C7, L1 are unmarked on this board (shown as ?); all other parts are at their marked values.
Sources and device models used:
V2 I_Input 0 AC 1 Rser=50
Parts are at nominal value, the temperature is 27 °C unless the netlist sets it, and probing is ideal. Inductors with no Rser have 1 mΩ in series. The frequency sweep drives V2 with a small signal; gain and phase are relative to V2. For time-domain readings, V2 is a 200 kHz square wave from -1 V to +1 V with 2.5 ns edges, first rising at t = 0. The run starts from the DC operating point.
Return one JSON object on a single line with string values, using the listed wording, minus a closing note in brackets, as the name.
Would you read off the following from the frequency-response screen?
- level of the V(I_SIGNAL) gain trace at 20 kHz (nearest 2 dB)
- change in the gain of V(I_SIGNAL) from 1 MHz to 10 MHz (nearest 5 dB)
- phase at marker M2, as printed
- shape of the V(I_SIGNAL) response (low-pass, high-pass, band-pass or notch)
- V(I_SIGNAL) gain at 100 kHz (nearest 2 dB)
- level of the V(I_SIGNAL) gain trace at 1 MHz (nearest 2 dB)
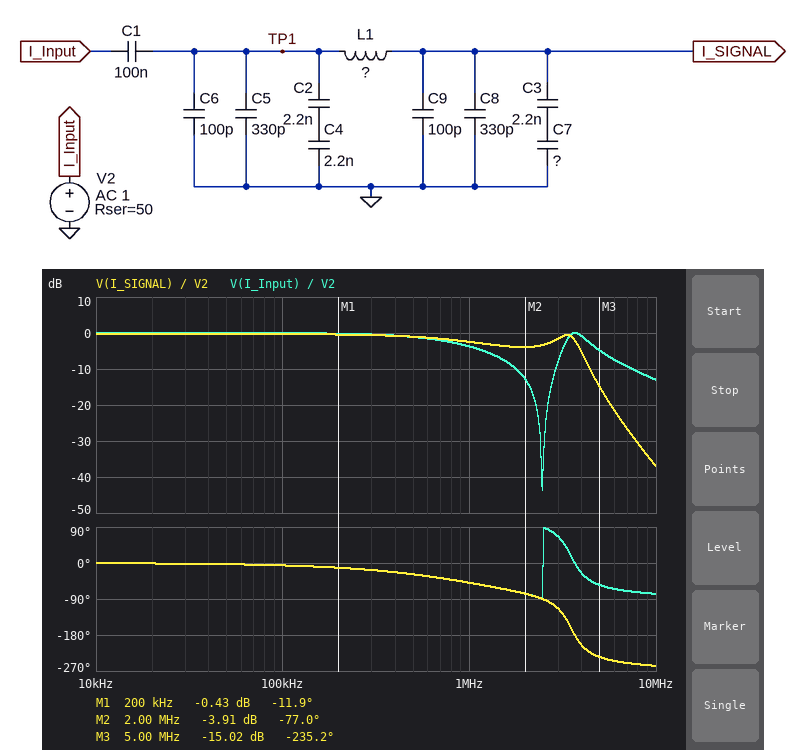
{"level of the V(I_SIGNAL) gain trace at 20 kHz": "0 dB", "change in the gain of V(I_SIGNAL) from 1 MHz to 10 MHz": "-35 dB", "phase at marker M2, as printed": "-77.0 deg", "shape of the V(I_SIGNAL) response": "low-pass", "V(I_SIGNAL) gain at 100 kHz": "0 dB", "level of the V(I_SIGNAL) gain trace at 1 MHz": "-2 dB"}
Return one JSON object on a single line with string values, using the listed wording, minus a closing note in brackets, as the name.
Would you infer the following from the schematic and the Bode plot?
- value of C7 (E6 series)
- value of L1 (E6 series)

{"value of C7": "4.7 nF", "value of L1": "2.2 µH"}
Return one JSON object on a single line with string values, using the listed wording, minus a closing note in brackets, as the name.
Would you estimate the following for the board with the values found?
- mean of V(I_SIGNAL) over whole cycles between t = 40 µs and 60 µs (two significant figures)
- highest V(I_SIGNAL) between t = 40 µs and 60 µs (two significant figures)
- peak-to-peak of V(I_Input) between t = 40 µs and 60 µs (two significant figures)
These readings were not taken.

{"mean of V(I_SIGNAL) over whole cycles between t = 40 µs and 60 µs": "970 mV", "highest V(I_SIGNAL) between t = 40 µs and 60 µs": "2.0 V", "peak-to-peak of V(I_Input) between t = 40 µs and 60 µs": "2.1 V"}
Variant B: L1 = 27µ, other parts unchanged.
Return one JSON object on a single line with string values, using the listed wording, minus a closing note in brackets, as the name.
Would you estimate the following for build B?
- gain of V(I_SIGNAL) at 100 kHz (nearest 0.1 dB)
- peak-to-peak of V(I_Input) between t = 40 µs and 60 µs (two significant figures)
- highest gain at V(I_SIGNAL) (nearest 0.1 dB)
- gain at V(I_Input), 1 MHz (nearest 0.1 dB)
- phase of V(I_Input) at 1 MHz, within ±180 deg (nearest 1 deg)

{"gain of V(I_SIGNAL) at 100 kHz": "-0.2 dB", "peak-to-peak of V(I_Input) between t = 40 µs and 60 µs": "2.6 V", "highest gain at V(I_SIGNAL)": "7.6 dB", "gain at V(I_Input), 1 MHz": "0 dB", "phase of V(I_Input) at 1 MHz, within ±180 deg": "5 deg"}
